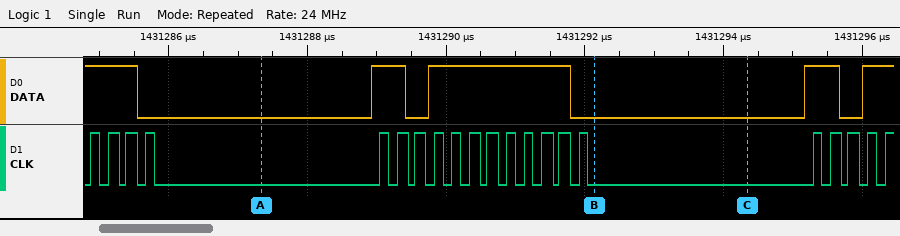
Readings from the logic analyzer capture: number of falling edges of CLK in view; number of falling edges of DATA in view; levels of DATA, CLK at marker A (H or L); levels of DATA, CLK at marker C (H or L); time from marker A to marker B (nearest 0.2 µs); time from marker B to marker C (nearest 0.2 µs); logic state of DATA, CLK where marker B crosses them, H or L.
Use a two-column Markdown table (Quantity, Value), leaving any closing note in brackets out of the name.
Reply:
| Quantity | Value |
|---|---|
| number of falling edges of CLK in view | 20 |
| number of falling edges of DATA in view | 4 |
| levels of DATA, CLK at marker A | DATA=L, CLK=L |
| levels of DATA, CLK at marker C | DATA=L, CLK=L |
| time from marker A to marker B | 4.8 µs |
| time from marker B to marker C | 2.2 µs |
| logic state of DATA, CLK where marker B crosses them, H or L | DATA=L, CLK=L |
